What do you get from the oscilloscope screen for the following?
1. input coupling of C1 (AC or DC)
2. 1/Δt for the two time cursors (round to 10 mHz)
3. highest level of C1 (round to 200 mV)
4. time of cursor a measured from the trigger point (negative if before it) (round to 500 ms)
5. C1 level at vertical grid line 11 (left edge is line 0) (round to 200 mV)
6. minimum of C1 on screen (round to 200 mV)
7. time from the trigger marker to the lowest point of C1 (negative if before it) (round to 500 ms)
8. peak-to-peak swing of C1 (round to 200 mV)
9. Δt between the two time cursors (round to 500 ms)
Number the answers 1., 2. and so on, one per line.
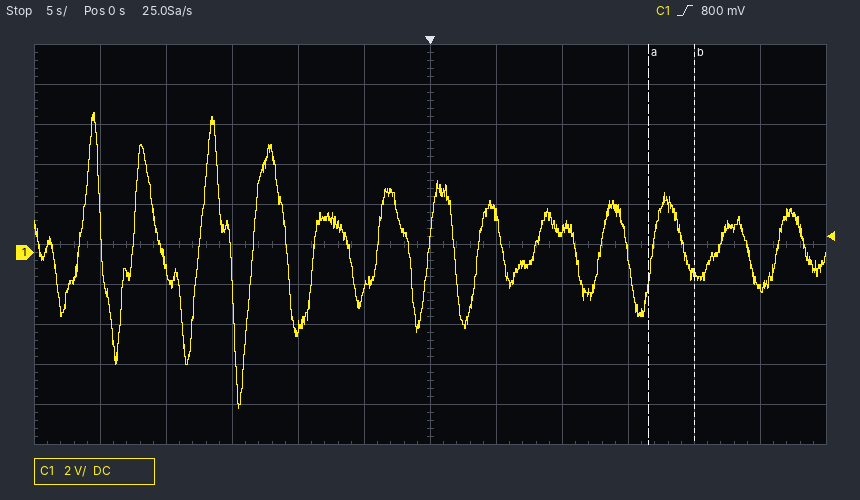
1. DC
2. 290 mHz
3. 7.0 V
4. +16.5 s
5. -1.8 V
6. -7.8 V
7. -14.5 s
8. 14.8 V
9. 3.5 s
